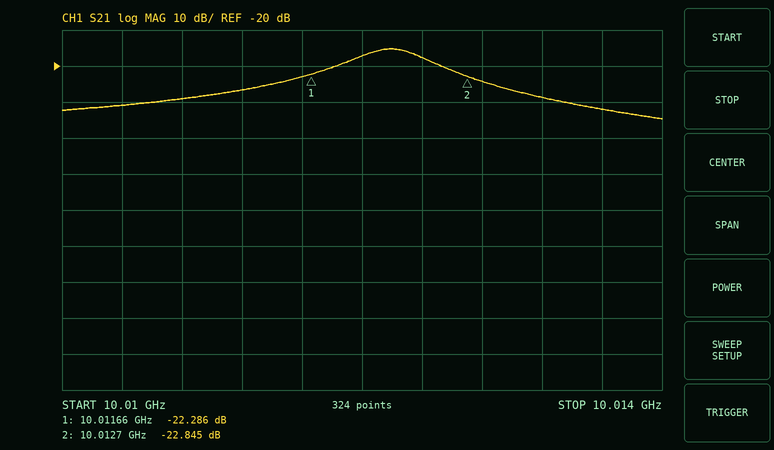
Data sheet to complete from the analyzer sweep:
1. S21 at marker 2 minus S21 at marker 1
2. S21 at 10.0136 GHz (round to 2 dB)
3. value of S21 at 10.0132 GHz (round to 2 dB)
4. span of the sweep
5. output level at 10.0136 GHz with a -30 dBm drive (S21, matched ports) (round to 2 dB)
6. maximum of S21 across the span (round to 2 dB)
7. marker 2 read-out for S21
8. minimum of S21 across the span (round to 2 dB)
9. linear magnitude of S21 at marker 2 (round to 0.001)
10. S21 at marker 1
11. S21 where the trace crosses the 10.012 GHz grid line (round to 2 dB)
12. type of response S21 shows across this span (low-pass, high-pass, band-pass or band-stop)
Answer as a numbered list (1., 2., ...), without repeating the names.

1. -0.559 dB
2. -32 dB
3. -28 dB
4. 4 MHz
5. -62 dBm
6. -16 dB
7. -22.845 dB
8. -34 dB
9. 0.072
10. -22.286 dB
11. -18 dB
12. band-pass
